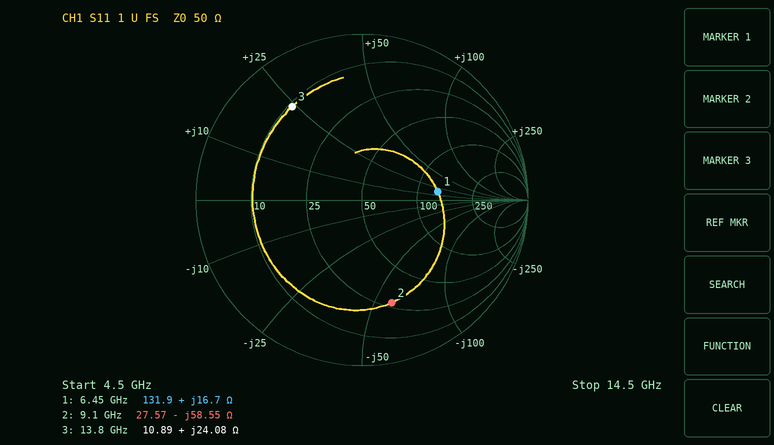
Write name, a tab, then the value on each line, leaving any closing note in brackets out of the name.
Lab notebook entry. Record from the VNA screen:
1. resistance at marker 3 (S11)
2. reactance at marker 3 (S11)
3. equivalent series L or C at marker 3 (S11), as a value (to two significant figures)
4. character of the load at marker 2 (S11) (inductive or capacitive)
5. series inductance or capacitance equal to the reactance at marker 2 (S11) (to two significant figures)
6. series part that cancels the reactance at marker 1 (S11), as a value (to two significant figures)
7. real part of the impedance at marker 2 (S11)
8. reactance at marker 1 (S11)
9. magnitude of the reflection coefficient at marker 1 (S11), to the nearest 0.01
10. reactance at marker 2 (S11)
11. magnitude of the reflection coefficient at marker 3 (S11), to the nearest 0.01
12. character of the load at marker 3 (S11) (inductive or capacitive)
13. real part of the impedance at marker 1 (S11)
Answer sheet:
resistance at marker 3	10.89 Ω
reactance at marker 3	+24.08 Ω
equivalent series L or C at marker 3 (S11), as a value	280 pH
character of the load at marker 2 (S11)	capacitive
series inductance or capacitance equal to the reactance at marker 2 (S11)	300 fF
series part that cancels the reactance at marker 1 (S11), as a value	1.5 pF
real part of the impedance at marker 2	27.57 Ω
reactance at marker 1	+16.7 Ω
magnitude of the reflection coefficient at marker 1 (S11), to the nearest 0.01	0.46
reactance at marker 2	-58.55 Ω
magnitude of the reflection coefficient at marker 3 (S11), to the nearest 0.01	0.70
character of the load at marker 3 (S11)	inductive
real part of the impedance at marker 1	131.9 Ω
